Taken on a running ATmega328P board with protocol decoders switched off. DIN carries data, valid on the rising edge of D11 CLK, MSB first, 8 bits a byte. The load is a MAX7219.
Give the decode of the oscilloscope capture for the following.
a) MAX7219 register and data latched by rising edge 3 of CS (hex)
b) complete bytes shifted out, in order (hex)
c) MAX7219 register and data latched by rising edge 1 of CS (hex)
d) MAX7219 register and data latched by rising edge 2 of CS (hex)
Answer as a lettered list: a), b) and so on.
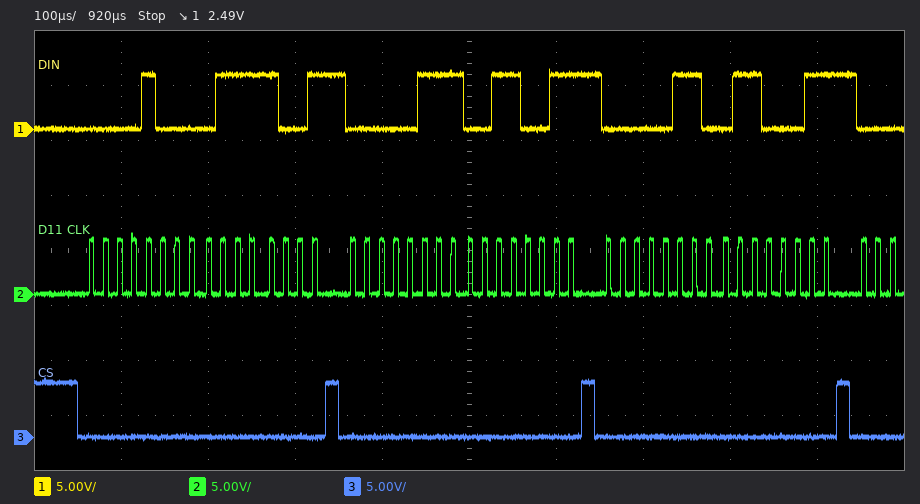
a) register 0x6, data 0x63
b) 0x08 0x79 0x07 0x33 0x06 0x63
c) register 0x8, data 0x79
d) register 0x7, data 0x33
